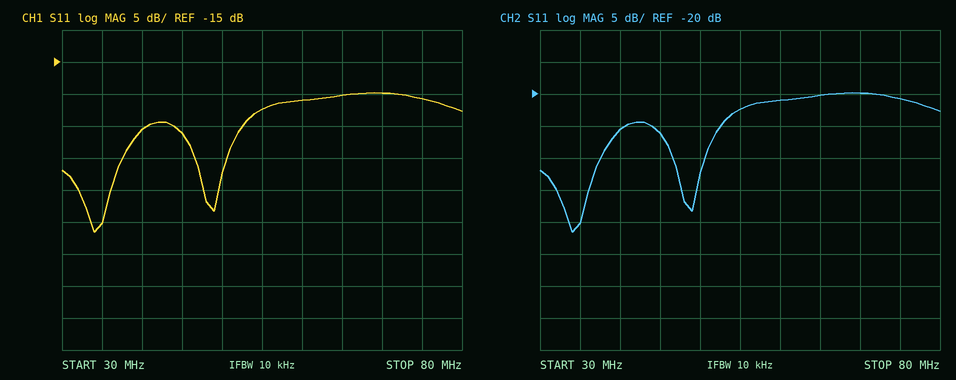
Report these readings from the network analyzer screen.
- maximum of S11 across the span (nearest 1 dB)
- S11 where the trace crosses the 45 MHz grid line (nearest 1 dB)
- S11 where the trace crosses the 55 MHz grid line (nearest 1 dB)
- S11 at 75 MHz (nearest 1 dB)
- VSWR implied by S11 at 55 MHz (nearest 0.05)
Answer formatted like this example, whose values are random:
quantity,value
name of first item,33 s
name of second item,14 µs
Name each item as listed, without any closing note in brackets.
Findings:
quantity,value
maximum of S11 across the span,-20 dB
S11 where the trace crosses the 45 MHz grid line,-26 dB
S11 where the trace crosses the 55 MHz grid line,-22 dB
S11 at 75 MHz,-21 dB
VSWR implied by S11 at 55 MHz,1.15
